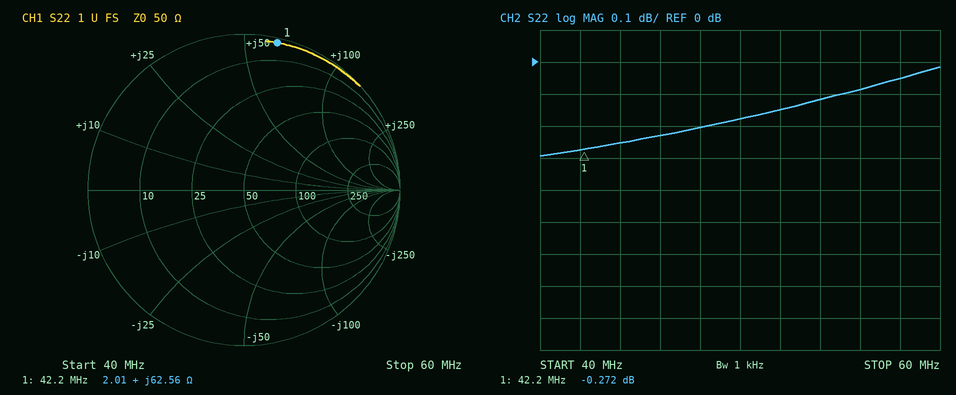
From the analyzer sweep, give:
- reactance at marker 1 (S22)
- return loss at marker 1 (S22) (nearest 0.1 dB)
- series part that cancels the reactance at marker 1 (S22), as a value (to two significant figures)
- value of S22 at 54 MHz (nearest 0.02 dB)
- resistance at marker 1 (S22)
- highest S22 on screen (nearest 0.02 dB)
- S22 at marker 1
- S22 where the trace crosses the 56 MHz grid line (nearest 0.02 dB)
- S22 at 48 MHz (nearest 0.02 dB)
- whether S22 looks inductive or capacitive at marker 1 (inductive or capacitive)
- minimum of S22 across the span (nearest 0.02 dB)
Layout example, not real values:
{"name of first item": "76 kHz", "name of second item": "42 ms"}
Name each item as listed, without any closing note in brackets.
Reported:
{"reactance at marker 1": "+62.56 Ω", "return loss at marker 1 (S22)": "0.3 dB", "series part that cancels the reactance at marker 1 (S22), as a value": "60 pF", "value of S22 at 54 MHz": "-0.12 dB", "resistance at marker 1": "2.01 Ω", "highest S22 on screen": "-0.02 dB", "S22 at marker 1": "-0.272 dB", "S22 where the trace crosses the 56 MHz grid line": "-0.08 dB", "S22 at 48 MHz": "-0.20 dB", "whether S22 looks inductive or capacitive at marker 1": "inductive", "minimum of S22 across the span": "-0.30 dB"}
